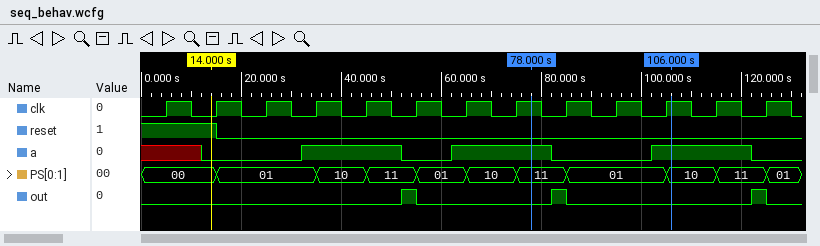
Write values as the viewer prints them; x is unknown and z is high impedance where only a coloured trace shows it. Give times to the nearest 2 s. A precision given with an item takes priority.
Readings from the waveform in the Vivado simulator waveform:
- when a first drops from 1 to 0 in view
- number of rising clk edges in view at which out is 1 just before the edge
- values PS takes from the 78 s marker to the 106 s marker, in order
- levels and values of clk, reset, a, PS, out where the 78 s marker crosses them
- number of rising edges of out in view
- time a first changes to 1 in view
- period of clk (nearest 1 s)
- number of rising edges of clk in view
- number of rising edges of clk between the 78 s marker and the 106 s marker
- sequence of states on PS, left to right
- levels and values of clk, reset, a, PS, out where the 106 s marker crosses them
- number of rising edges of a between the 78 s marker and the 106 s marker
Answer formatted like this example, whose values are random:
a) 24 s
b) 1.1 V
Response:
a) 52 s
b) 3
c) 11, 01, 10
d) clk=1, reset=0, a=1, PS=11, out=0
e) 3
f) 32 s
g) 10 s
h) 13
i) 3
j) 00, 01, 10, 11, 01, 10, 11, 01, 10, 11, 01
k) clk=1, reset=0, a=1, PS=10, out=0
l) 1
